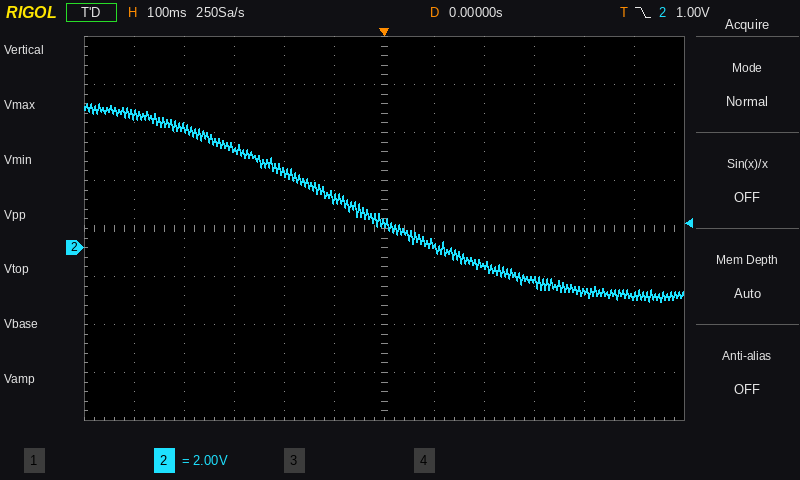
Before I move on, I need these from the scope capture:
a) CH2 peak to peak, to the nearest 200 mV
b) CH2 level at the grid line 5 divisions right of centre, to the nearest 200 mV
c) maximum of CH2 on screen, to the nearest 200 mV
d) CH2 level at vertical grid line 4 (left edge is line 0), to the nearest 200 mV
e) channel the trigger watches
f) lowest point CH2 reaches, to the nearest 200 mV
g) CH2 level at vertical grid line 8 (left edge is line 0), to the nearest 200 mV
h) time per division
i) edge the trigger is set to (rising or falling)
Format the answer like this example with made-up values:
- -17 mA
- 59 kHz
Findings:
- 8.2 V
- -2.0 V
- 6.0 V
- 3.2 V
- CH2
- -2.2 V
- -800 mV
- 100 ms
- falling
